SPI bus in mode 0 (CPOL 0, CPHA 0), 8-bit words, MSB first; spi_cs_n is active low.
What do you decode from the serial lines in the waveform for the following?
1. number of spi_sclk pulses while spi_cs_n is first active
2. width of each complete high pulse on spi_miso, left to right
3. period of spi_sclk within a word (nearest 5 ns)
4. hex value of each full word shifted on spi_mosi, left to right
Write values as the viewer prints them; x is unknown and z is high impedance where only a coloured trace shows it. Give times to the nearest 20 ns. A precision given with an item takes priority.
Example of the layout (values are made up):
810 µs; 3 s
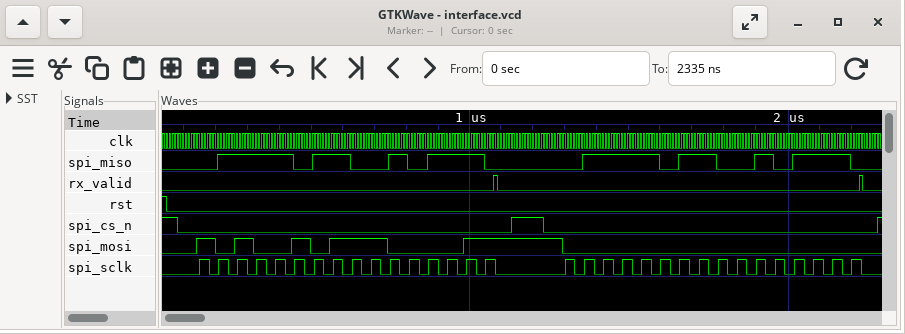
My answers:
16; 240 ns, 120 ns, 60 ns, 180 ns, 240 ns, 120 ns, 60 ns, 180 ns; 60 ns; A5, C3, 00, 00
